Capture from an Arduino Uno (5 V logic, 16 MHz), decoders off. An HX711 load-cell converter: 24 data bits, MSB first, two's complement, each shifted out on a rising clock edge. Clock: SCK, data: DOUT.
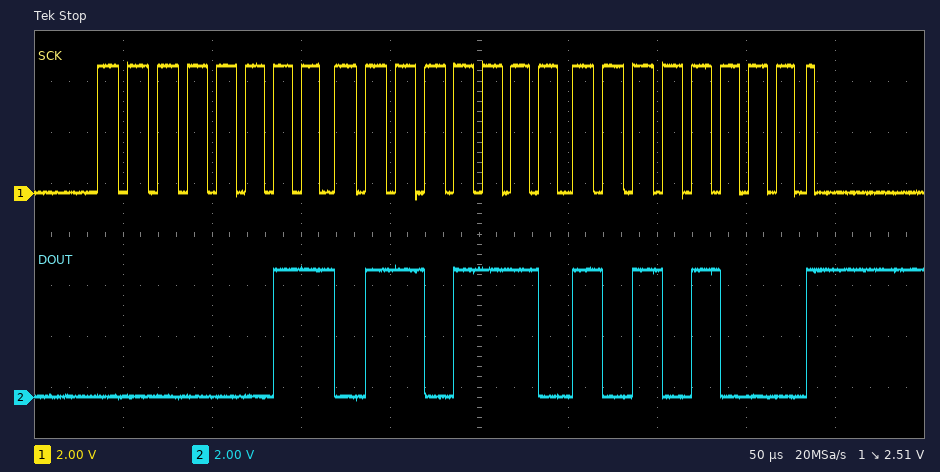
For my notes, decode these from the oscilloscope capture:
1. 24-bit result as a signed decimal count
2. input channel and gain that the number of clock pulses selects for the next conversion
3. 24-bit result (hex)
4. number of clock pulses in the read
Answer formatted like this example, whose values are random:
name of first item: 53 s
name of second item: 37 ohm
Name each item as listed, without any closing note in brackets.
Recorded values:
24-bit result as a signed decimal count: 224936
input channel and gain that the number of clock pulses selects for the next conversion: channel A, gain 128
24-bit result: 0x036EA8
number of clock pulses in the read: 25
